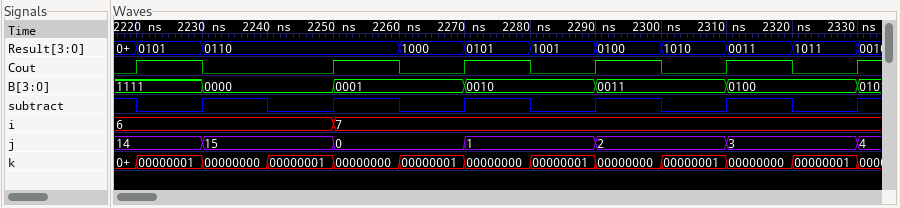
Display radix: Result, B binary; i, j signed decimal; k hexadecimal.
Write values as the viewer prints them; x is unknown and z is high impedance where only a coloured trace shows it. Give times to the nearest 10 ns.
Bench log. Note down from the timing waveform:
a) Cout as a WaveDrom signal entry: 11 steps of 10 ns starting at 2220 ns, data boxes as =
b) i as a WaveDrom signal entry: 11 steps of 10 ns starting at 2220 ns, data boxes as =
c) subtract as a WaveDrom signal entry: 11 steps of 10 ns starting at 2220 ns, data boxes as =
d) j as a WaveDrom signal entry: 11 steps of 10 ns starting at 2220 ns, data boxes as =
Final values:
{name: 'Cout', wave: '10.10101010'}
{name: 'i', wave: '=..=.......', data: '6 7'}
{name: 'subtract', wave: '01010101010'}
{name: 'j', wave: '==.=.=.=.=.', data: '14 15 0 1 2 3'}
